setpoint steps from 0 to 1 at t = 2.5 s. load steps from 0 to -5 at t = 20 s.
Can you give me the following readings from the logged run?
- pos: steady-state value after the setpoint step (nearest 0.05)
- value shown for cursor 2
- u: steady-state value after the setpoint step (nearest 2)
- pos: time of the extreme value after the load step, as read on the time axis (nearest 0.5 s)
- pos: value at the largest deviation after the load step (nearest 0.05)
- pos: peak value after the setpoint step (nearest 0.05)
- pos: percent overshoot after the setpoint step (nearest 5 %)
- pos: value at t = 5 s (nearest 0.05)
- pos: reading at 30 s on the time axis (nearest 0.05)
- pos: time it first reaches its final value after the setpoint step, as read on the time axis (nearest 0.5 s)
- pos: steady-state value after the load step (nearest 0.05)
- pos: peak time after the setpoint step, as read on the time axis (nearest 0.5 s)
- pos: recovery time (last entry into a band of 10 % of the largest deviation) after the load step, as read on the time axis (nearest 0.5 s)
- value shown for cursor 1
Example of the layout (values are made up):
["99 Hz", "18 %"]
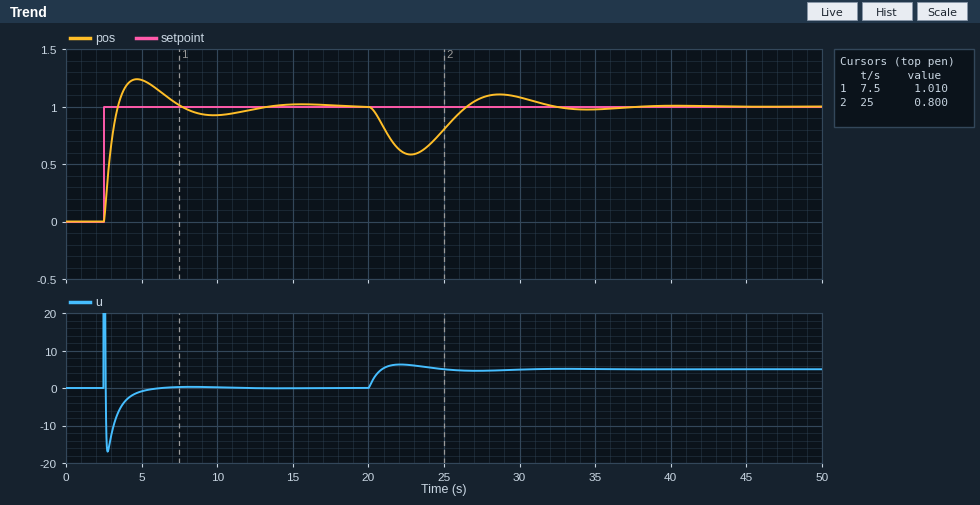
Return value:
["1.00", "0.800", "0", "23.0 s", "0.60", "1.25", "25 %", "1.25", "1.10", "3.5 s", "1.00", "4.5 s", "31.0 s", "1.010"]
